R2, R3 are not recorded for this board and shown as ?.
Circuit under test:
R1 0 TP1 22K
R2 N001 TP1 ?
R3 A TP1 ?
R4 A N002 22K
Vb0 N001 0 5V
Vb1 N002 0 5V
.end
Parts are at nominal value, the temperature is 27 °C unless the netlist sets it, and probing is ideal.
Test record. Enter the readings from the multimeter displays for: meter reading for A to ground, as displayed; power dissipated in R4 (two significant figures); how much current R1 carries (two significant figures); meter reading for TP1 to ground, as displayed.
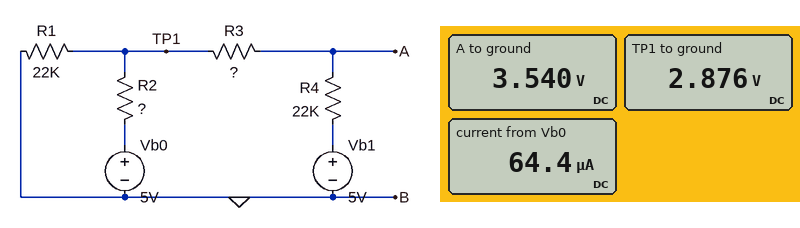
3.540 V
97 µW
130 µA
2.876 V
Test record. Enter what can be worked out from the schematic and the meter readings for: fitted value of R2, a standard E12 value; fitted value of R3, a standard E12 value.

33 kΩ
10 kΩ
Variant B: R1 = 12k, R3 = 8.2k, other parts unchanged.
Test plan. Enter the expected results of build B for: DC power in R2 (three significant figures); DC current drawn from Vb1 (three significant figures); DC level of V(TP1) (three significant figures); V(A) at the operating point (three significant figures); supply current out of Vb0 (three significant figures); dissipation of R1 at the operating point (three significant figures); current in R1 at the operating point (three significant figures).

244 µW
94.0 µA
2.16 V
2.93 V
86.0 µA
389 µW
180 µA
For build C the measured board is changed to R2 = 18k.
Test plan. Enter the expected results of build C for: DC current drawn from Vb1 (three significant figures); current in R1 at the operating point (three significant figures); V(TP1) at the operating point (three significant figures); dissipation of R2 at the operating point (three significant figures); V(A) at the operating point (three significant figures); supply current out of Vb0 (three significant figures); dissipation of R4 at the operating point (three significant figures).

53.7 µA
149 µA
3.28 V
164 µW
3.82 V
95.5 µA
63.4 µW
